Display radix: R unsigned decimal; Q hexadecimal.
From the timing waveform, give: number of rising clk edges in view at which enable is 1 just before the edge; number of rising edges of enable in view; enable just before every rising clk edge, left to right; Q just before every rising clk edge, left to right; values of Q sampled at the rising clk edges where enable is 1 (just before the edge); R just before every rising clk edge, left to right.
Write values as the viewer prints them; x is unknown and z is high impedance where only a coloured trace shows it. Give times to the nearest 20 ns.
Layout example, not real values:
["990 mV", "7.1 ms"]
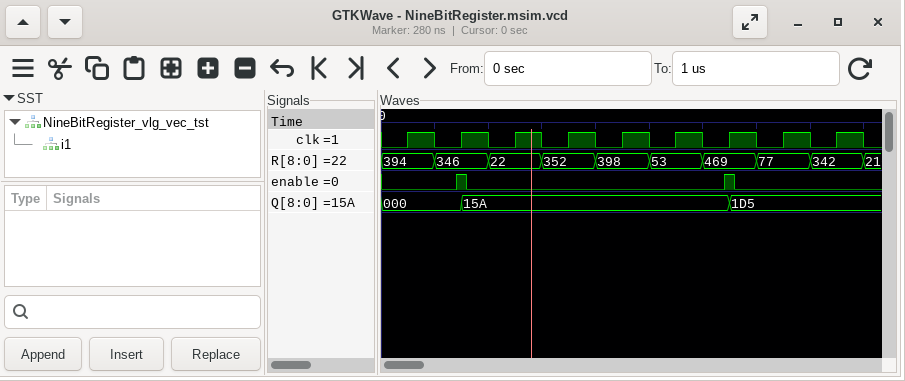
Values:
["2", "2", "0 1 0 0 0 0 1 0 0", "000, 000, 15A, 15A, 15A, 15A, 15A, 1D5, 1D5", "000, 15A", "394, 346, 22, 352, 398, 53, 469, 77, 342"]
